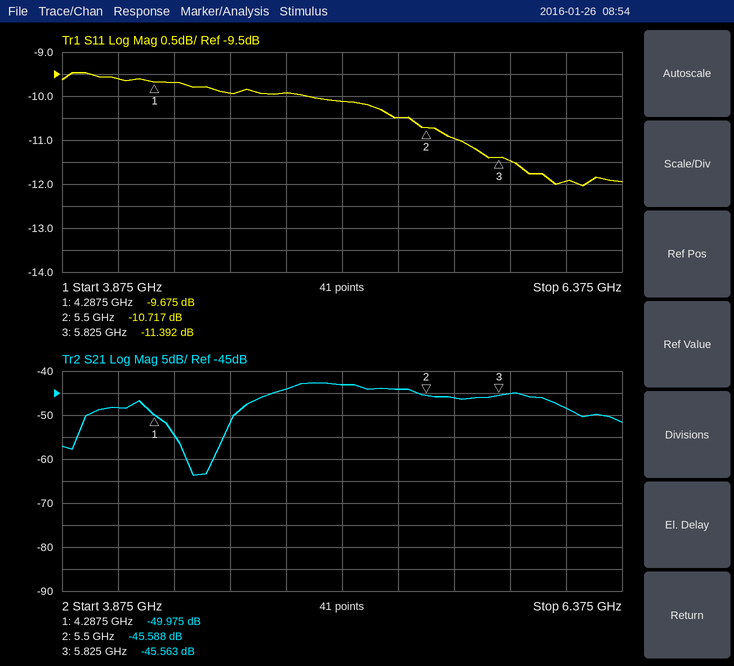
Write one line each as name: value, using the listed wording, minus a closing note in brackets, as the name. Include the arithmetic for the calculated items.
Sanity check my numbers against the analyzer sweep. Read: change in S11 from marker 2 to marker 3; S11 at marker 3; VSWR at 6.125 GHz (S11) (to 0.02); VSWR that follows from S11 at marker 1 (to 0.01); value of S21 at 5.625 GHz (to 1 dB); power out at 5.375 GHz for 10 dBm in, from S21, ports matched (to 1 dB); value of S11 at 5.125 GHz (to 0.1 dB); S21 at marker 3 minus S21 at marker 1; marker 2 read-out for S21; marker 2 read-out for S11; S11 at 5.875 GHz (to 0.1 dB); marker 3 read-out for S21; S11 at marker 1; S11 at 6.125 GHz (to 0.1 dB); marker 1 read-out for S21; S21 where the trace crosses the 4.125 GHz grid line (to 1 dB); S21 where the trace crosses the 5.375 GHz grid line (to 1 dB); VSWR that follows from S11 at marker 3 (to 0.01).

change in S11 from marker 2 to marker 3: -11.392 − (-10.717) = -0.675 dB
S11 at marker 3: -11.392 dB
VSWR at 6.125 GHz (S11): |Γ| = 10^(-11.9/20) = 0.2541; VSWR = (1 + 0.2541)/(1 − 0.2541) ≈ 1.68
VSWR that follows from S11 at marker 1: (1 + 0.3283)/(1 − 0.3283) ≈ 1.98
value of S21 at 5.625 GHz: -46 dB
power out at 5.375 GHz for 10 dBm in, from S21, ports matched: 10 dBm + (-44 dB) = -34 dBm
value of S11 at 5.125 GHz: -10.1 dB
S21 at marker 3 minus S21 at marker 1: -45.563 − (-49.975) = 4.412 dB
marker 2 read-out for S21: -45.588 dB
marker 2 read-out for S11: -10.717 dB
S11 at 5.875 GHz: -11.5 dB
marker 3 read-out for S21: -45.563 dB
S11 at marker 1: -9.675 dB
S11 at 6.125 GHz: -11.9 dB
marker 1 read-out for S21: -49.975 dB
S21 where the trace crosses the 4.125 GHz grid line: -48 dB
S21 where the trace crosses the 5.375 GHz grid line: -44 dB
VSWR that follows from S11 at marker 3: (1 + 0.2694)/(1 − 0.2694) ≈ 1.74
